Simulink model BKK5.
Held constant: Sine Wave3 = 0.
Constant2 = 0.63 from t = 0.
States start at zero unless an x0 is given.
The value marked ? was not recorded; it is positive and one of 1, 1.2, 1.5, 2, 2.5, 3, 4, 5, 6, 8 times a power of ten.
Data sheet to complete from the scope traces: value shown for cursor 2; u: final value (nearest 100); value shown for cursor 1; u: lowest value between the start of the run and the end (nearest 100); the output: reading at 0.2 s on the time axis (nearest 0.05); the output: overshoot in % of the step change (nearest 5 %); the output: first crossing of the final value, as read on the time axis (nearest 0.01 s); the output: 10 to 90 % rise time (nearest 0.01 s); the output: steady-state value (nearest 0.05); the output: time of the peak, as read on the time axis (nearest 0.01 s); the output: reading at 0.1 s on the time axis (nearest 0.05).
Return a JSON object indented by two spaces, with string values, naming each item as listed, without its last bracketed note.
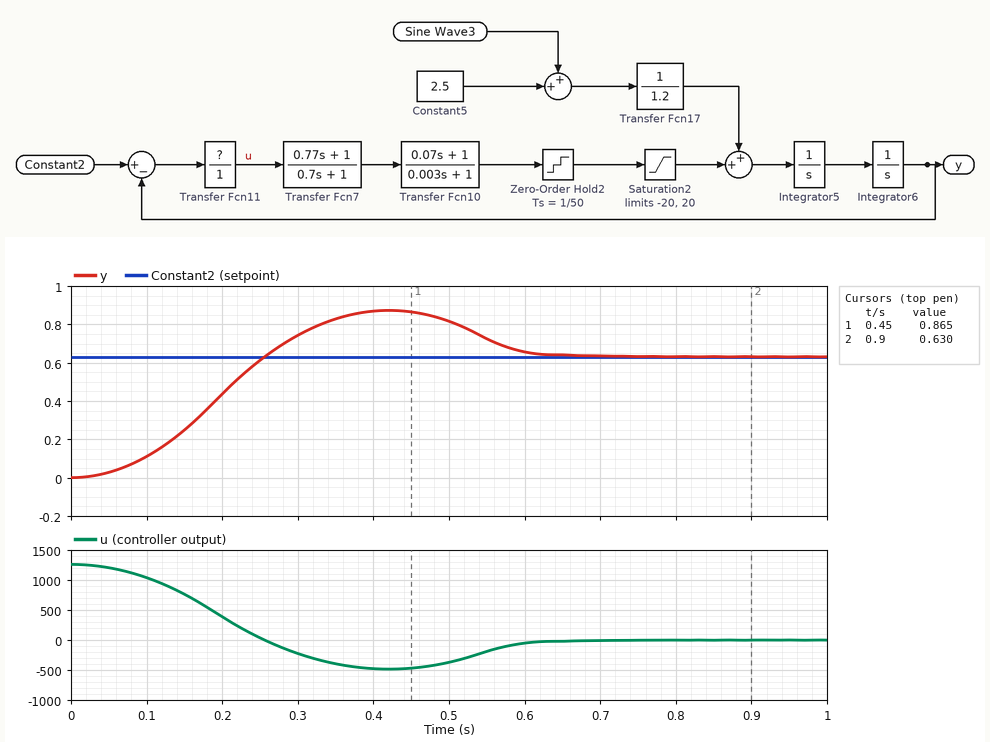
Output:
{
  "value shown for cursor 2": "0.630",
  "u: final value": "0",
  "value shown for cursor 1": "0.865",
  "u: lowest value between the start of the run and the end": "-500",
  "the output: reading at 0.2 s on the time axis": "0.45",
  "the output: overshoot in % of the step change": "40 %",
  "the output: first crossing of the final value, as read on the time axis": "0.26 s",
  "the output: 10 to 90 % rise time": "0.16 s",
  "the output: steady-state value": "0.65",
  "the output: time of the peak, as read on the time axis": "0.42 s",
  "the output: reading at 0.1 s on the time axis": "0.10"
}
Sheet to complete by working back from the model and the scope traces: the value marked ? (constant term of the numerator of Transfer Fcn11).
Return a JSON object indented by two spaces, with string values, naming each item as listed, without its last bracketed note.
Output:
{
  "the value marked ?": "2000"
}
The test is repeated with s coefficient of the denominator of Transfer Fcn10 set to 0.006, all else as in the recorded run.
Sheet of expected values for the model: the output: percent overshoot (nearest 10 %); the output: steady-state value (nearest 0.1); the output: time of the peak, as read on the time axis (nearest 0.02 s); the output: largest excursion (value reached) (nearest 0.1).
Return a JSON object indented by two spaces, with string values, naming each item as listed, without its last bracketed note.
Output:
{
  "the output: percent overshoot": "60 %",
  "the output: steady-state value": "0.6",
  "the output: time of the peak, as read on the time axis": "0.44 s",
  "the output: largest excursion (value reached)": "1.0"
}
